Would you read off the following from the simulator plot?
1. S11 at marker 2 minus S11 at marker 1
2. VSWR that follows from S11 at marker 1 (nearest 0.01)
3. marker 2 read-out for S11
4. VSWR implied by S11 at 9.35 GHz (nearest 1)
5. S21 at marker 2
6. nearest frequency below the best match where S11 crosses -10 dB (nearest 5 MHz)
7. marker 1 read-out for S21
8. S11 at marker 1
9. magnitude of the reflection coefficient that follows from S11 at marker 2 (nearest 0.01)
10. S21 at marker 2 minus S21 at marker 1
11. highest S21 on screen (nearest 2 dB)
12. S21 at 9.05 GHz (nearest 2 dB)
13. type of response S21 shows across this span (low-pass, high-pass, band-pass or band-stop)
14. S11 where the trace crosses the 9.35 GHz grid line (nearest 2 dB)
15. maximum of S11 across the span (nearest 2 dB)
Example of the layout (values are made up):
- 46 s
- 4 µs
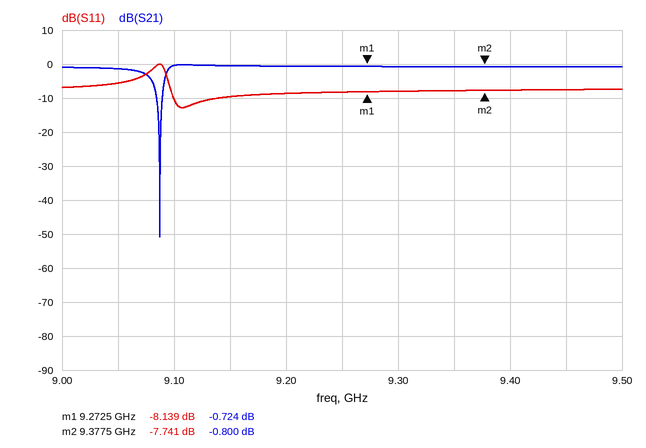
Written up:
- 0.398 dB
- 2.29
- -7.741 dB
- 2
- -0.800 dB
- 9.100 GHz
- -0.724 dB
- -8.139 dB
- 0.41
- -0.076 dB
- 0 dB
- -2 dB
- band-stop
- -8 dB
- 0 dB
